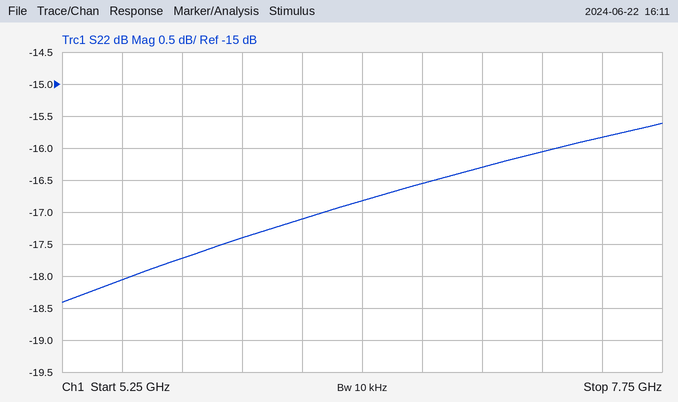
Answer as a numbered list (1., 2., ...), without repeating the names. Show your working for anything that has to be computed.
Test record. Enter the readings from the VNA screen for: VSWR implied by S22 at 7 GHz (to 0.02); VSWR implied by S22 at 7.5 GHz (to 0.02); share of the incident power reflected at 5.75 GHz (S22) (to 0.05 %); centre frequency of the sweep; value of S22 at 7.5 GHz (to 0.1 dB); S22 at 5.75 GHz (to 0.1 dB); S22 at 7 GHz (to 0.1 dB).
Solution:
1. |Γ| = 10^(-16.3/20) = 0.1531; VSWR = (1 + 0.1531)/(1 − 0.1531) ≈ 1.36
2. |Γ| = 10^(-15.8/20) = 0.1622; VSWR = (1 + 0.1622)/(1 − 0.1622) ≈ 1.39, so 1.38 to the nearest 0.02
3. 10^(-17.7/10) ≈ 1.70 %
4. 6.5 GHz
5. -15.8 dB
6. -17.7 dB
7. -16.3 dB
